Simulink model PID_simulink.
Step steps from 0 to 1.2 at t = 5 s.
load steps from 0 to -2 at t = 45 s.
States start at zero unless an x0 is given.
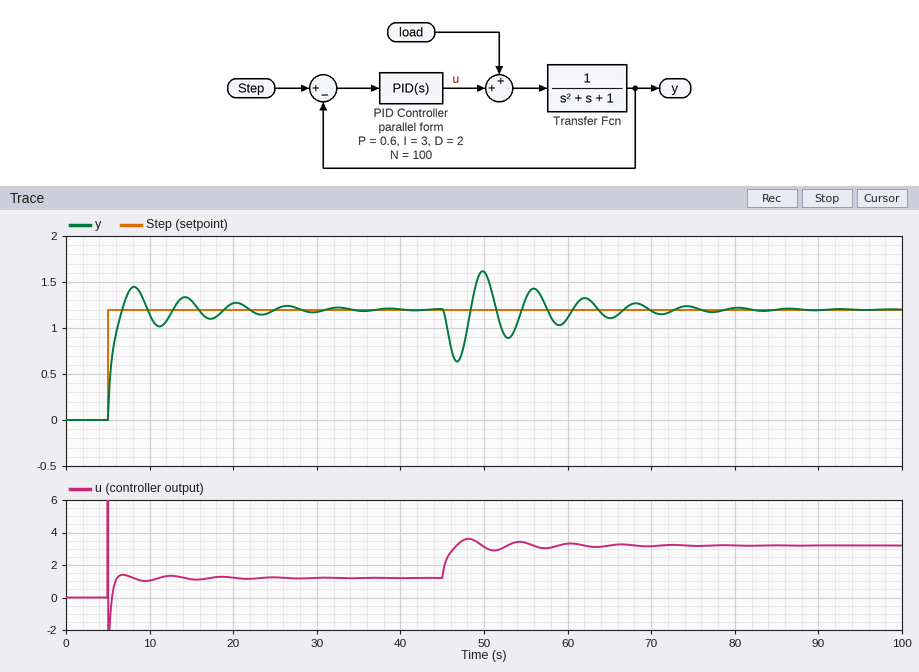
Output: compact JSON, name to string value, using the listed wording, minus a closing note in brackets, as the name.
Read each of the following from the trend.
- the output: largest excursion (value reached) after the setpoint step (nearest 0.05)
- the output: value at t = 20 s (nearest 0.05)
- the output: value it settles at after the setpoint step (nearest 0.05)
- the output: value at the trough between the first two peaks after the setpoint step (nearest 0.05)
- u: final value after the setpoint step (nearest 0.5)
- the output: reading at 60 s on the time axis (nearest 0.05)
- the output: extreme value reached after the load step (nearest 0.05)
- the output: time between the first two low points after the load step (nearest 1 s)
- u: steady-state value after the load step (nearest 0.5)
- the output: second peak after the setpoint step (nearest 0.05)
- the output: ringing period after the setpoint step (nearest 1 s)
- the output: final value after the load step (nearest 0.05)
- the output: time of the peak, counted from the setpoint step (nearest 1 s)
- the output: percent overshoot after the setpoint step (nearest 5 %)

{"the output: largest excursion (value reached) after the setpoint step": "1.45", "the output: value at t = 20 s": "1.25", "the output: value it settles at after the setpoint step": "1.20", "the output: value at the trough between the first two peaks after the setpoint step": "1.00", "u: final value after the setpoint step": "1.0", "the output: reading at 60 s on the time axis": "1.10", "the output: extreme value reached after the load step": "0.65", "the output: time between the first two low points after the load step": "6 s", "u: steady-state value after the load step": "3.0", "the output: second peak after the setpoint step": "1.35", "the output: ringing period after the setpoint step": "6 s", "the output: final value after the load step": "1.20", "the output: time of the peak, counted from the setpoint step": "3 s", "the output: percent overshoot after the setpoint step": "20 %"}
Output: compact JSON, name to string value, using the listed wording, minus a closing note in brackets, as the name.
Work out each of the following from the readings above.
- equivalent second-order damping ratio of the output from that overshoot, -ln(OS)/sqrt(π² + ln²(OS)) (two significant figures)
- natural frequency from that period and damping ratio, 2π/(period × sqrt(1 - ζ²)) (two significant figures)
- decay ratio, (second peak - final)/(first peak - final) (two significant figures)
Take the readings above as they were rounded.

{"equivalent second-order damping ratio of the output from that overshoot, -ln(OS)/sqrt(π² + ln²(OS))": "0.46", "natural frequency from that period and damping ratio, 2π/(period × sqrt(1 - ζ²))": "1.2 rad/s", "decay ratio, (second peak - final)/(first peak - final)": "0.60"}
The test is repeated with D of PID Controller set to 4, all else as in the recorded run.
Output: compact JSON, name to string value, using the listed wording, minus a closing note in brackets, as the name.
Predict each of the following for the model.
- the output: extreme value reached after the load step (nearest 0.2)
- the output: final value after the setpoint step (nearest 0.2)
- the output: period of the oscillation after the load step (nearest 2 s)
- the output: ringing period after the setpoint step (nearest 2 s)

{"the output: extreme value reached after the load step": "0.8", "the output: final value after the setpoint step": "1.2", "the output: period of the oscillation after the load step": "8 s", "the output: ringing period after the setpoint step": "8 s"}
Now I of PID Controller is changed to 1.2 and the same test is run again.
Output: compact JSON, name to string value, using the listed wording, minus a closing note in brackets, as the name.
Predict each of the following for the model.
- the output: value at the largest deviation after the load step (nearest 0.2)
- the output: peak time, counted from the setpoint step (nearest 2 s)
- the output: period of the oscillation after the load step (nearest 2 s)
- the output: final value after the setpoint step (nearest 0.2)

{"the output: value at the largest deviation after the load step": "0.4", "the output: peak time, counted from the setpoint step": "6 s", "the output: period of the oscillation after the load step": "10 s", "the output: final value after the setpoint step": "1.2"}
